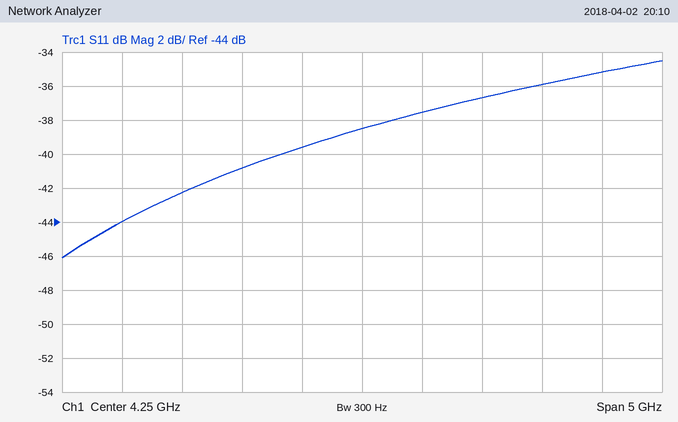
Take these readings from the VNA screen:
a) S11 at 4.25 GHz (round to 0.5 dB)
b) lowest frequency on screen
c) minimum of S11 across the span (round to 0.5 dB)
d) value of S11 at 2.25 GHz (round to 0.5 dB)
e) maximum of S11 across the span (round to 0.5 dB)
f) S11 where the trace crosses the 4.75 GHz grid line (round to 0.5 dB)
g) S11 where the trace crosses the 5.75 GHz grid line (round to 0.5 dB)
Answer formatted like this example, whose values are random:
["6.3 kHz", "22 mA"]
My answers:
["-38.5 dB", "1.75 GHz", "-46.0 dB", "-44.0 dB", "-34.5 dB", "-37.5 dB", "-36.0 dB"]
